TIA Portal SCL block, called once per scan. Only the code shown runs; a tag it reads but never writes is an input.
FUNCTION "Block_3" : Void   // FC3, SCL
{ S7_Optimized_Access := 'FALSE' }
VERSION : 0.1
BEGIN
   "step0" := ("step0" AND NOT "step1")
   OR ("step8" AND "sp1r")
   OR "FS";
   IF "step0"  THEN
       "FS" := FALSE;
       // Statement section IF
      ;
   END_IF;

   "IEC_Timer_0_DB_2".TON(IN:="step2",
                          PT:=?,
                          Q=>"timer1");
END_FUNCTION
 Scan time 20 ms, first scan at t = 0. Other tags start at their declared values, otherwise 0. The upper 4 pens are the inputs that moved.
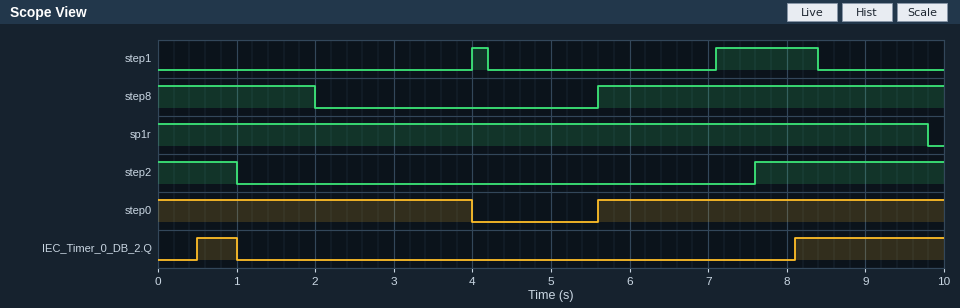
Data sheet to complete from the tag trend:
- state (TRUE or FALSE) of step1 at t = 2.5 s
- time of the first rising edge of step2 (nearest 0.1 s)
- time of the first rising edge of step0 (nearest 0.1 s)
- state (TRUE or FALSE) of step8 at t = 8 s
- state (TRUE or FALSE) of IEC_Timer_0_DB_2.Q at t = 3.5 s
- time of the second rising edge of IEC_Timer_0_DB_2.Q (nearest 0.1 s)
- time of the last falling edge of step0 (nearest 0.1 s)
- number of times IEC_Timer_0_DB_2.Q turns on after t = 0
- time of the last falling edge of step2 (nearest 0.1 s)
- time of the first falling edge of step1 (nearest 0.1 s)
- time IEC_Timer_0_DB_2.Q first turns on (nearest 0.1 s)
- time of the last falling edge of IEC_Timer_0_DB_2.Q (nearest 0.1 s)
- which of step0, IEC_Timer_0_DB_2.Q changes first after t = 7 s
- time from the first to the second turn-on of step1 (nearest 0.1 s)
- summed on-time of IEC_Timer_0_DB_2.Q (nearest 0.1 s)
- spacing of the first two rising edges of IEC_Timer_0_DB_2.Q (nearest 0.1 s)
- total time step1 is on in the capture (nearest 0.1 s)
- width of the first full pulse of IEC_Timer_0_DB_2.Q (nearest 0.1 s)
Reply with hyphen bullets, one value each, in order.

- FALSE
- 7.6 s
- 5.6 s
- TRUE
- FALSE
- 8.1 s
- 4.0 s
- 2
- 1.0 s
- 4.2 s
- 0.5 s
- 1.0 s
- IEC_Timer_0_DB_2.Q
- 3.1 s
- 2.4 s
- 7.6 s
- 1.5 s
- 0.5 s
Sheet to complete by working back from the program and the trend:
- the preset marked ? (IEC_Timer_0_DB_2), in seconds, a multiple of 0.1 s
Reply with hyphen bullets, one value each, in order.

- 0.5 s
